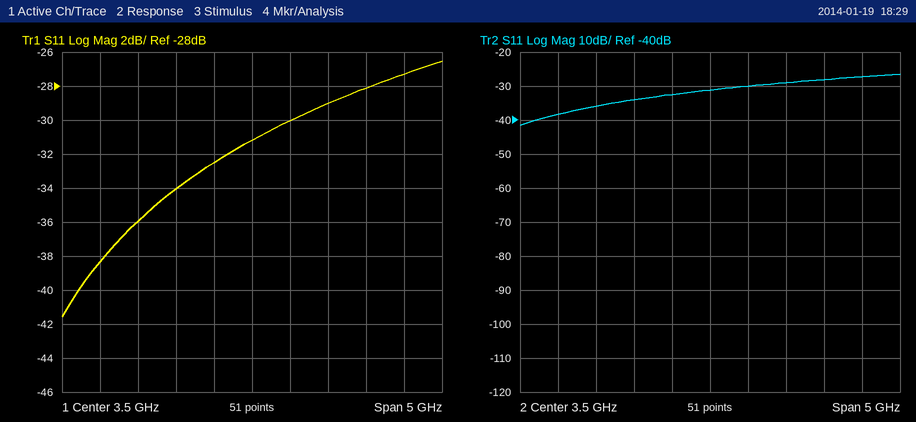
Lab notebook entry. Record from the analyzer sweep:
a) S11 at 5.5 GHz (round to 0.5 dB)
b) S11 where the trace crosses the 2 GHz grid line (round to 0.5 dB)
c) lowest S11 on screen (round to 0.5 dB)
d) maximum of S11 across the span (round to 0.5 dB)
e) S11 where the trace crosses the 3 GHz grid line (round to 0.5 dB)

-27.5 dB
-36.0 dB
-41.5 dB
-26.5 dB
-32.5 dB
